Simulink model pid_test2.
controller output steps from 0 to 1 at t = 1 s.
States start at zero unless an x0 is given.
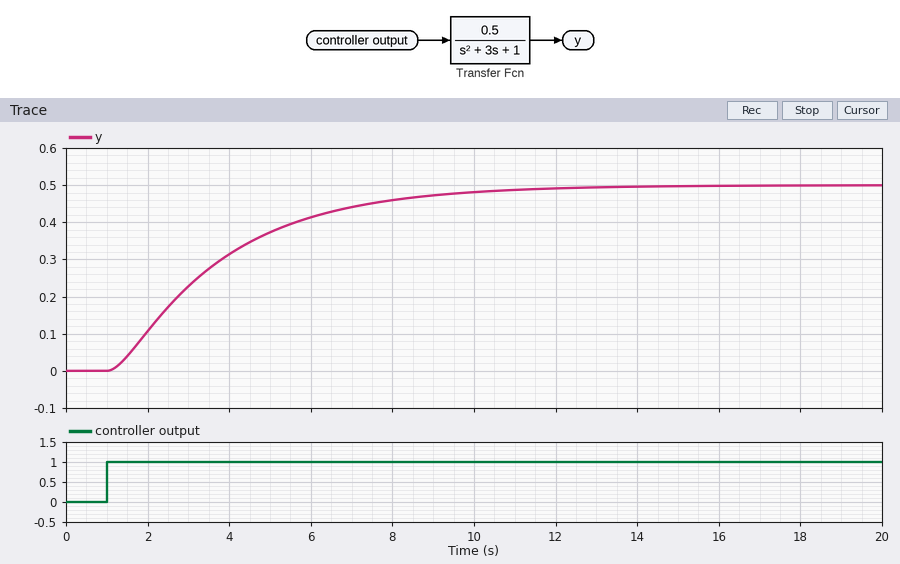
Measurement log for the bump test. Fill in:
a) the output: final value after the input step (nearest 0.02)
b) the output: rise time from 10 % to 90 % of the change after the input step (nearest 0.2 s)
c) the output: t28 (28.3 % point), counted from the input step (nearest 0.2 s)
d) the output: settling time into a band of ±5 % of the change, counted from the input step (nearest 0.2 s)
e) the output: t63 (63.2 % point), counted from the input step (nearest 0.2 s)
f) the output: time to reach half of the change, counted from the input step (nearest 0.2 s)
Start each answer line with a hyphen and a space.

- 0.50
- 5.8 s
- 1.2 s
- 8.2 s
- 3.0 s
- 2.2 s
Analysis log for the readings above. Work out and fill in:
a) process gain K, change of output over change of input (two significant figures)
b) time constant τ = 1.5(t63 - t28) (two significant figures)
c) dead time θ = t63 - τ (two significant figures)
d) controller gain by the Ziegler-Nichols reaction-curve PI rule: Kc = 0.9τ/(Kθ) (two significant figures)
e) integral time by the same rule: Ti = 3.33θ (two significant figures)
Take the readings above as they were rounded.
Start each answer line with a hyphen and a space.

- 0.50
- 2.7 s
- 0.30 s
- 16
- 1.00 s
